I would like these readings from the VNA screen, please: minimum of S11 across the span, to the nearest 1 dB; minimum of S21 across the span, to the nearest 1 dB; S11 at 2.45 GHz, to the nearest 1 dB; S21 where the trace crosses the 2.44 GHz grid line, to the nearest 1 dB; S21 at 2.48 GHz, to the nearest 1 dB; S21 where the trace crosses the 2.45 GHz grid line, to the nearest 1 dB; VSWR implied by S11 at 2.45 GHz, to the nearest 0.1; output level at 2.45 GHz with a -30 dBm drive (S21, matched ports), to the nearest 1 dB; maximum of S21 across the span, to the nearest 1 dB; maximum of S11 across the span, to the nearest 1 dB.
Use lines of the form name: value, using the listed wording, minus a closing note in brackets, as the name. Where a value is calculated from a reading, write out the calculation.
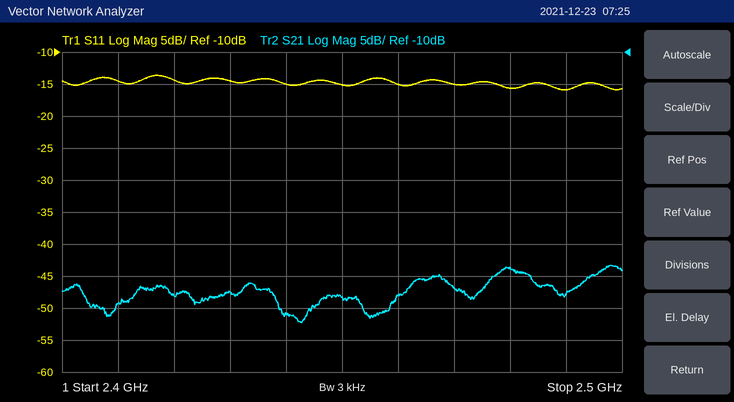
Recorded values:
minimum of S11 across the span, to the nearest 1 dB: -16 dB
minimum of S21 across the span, to the nearest 1 dB: -52 dB
S11 at 2.45 GHz, to the nearest 1 dB: -15 dB
S21 where the trace crosses the 2.44 GHz grid line, to the nearest 1 dB: -51 dB
S21 at 2.48 GHz, to the nearest 1 dB: -44 dB
S21 where the trace crosses the 2.45 GHz grid line, to the nearest 1 dB: -48 dB
VSWR implied by S11 at 2.45 GHz, to the nearest 0.1: |Γ| = 10^(-15/20) = 0.1778; VSWR = (1 + 0.1778)/(1 − 0.1778) ≈ 1.4
output level at 2.45 GHz with a -30 dBm drive (S21, matched ports), to the nearest 1 dB: -30 dBm + (-48 dB) = -78 dBm
maximum of S21 across the span, to the nearest 1 dB: -43 dB
maximum of S11 across the span, to the nearest 1 dB: -14 dB
